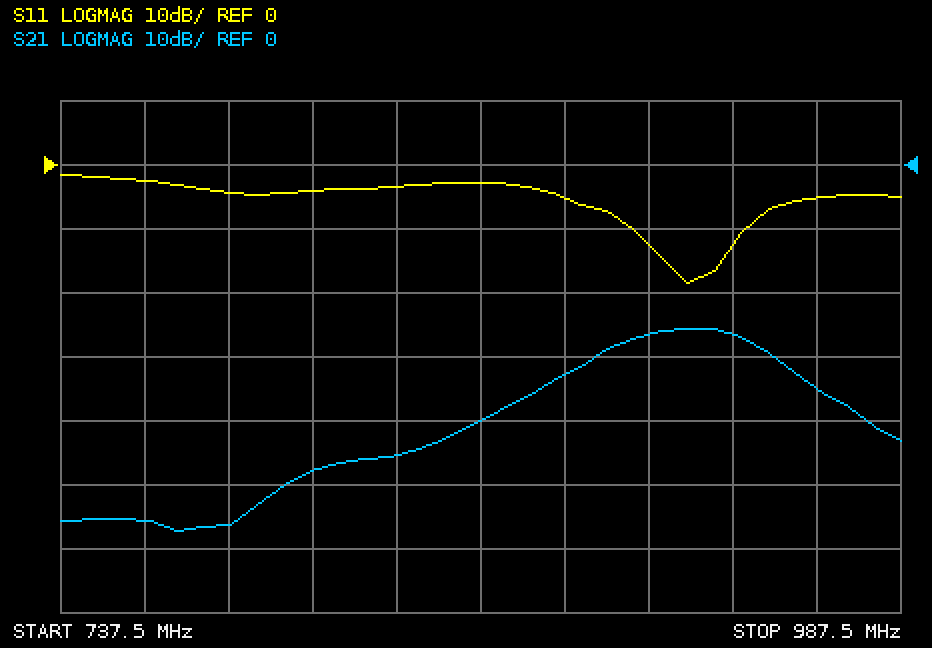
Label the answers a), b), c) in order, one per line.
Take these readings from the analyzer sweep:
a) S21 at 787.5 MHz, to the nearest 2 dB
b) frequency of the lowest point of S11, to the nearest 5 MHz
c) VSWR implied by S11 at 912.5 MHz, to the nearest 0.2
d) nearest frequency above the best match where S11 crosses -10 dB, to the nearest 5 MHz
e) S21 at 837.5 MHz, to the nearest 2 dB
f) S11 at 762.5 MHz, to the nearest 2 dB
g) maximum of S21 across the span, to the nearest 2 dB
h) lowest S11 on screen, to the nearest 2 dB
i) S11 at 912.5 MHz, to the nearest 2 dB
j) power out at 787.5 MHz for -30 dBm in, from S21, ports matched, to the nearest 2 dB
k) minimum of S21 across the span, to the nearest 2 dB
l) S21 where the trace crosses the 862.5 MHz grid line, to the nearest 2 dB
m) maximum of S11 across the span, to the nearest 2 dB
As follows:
a) -56 dB
b) 925 MHz
c) 1.6
d) 940 MHz
e) -46 dB
f) -2 dB
g) -26 dB
h) -18 dB
i) -12 dB
j) -86 dBm
k) -58 dB
l) -40 dB
m) -2 dB
